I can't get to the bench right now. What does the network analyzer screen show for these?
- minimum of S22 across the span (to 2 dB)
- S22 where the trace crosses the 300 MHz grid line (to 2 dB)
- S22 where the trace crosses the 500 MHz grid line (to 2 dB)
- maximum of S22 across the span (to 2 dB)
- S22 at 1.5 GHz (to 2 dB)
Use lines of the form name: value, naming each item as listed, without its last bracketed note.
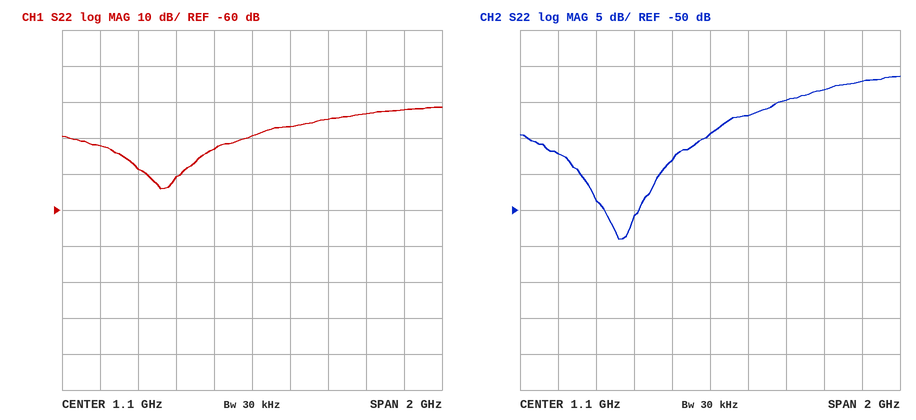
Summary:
minimum of S22 across the span: -54 dB
S22 where the trace crosses the 300 MHz grid line: -42 dB
S22 where the trace crosses the 500 MHz grid line: -48 dB
maximum of S22 across the span: -32 dB
S22 at 1.5 GHz: -34 dB
